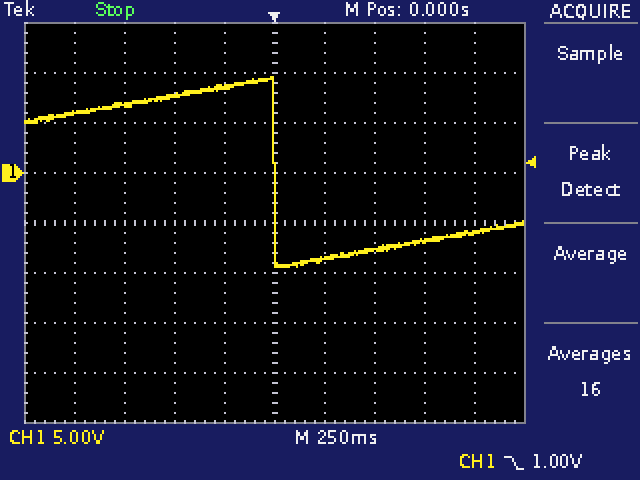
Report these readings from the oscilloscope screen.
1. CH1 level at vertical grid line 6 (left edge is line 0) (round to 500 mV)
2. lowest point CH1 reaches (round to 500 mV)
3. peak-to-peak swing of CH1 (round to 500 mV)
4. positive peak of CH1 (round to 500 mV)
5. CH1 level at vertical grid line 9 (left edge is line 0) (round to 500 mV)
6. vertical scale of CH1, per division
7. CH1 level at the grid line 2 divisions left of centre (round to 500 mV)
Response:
-8.5 V
-9.5 V
19.0 V
9.5 V
-6.0 V
5 V
8.0 V
